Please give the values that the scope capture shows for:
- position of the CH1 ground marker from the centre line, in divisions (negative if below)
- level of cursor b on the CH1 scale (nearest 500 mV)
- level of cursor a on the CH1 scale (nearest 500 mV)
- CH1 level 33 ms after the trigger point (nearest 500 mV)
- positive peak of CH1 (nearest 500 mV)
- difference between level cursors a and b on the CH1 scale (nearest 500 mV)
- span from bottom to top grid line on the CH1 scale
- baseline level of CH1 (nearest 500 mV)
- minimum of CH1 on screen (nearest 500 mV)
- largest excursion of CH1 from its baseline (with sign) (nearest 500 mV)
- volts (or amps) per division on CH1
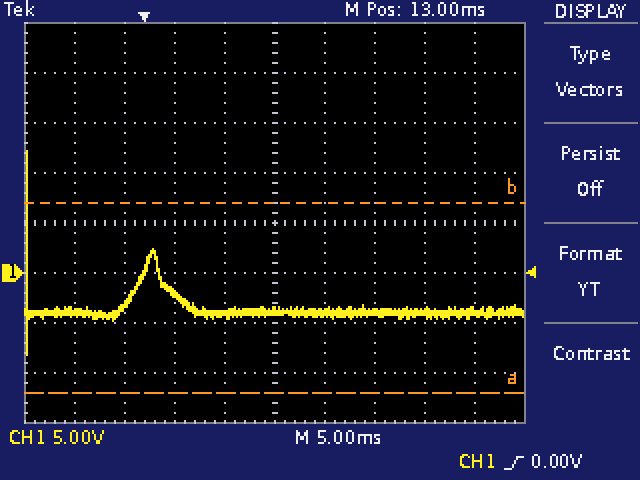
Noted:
-1.0 div
7.0 V
-12.0 V
-4.0 V
12.0 V
19.0 V
40 V
-4.0 V
-8.0 V
+16.0 V
5 V
